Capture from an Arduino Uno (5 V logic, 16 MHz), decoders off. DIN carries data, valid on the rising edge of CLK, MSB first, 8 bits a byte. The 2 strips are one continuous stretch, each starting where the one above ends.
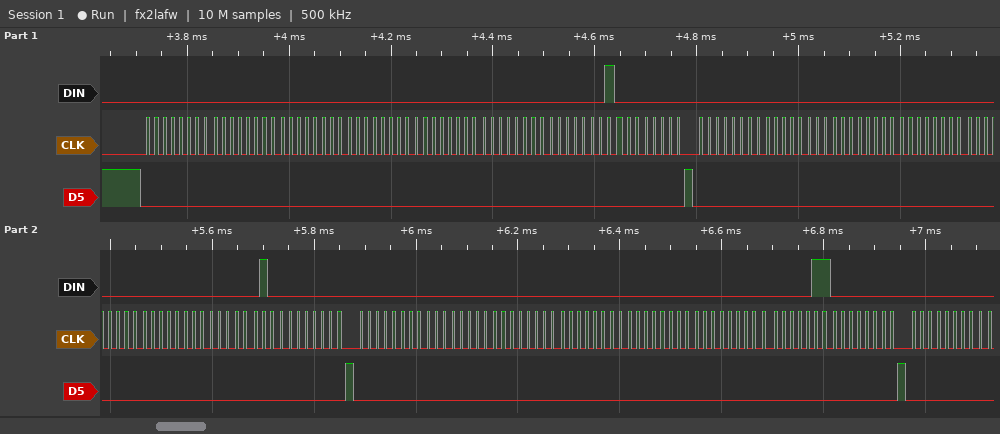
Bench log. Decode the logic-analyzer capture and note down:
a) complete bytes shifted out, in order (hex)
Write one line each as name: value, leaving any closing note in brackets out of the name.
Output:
complete bytes shifted out, in order: 00 00 00 00 00 00 01 00 00 00 00 00 00 00 02 00 00 00 00 00 00 00 03 00 00
